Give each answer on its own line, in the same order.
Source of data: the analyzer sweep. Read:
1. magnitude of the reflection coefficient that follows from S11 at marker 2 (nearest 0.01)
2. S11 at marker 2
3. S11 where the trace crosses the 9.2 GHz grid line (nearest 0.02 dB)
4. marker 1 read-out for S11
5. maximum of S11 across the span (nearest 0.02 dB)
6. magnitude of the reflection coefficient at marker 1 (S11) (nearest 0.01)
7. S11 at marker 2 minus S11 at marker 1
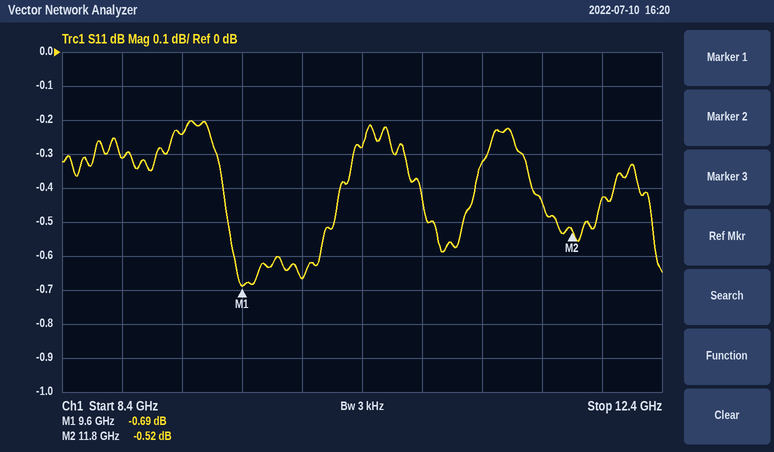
0.94
-0.52 dB
-0.24 dB
-0.69 dB
-0.20 dB
0.92
0.17 dB
